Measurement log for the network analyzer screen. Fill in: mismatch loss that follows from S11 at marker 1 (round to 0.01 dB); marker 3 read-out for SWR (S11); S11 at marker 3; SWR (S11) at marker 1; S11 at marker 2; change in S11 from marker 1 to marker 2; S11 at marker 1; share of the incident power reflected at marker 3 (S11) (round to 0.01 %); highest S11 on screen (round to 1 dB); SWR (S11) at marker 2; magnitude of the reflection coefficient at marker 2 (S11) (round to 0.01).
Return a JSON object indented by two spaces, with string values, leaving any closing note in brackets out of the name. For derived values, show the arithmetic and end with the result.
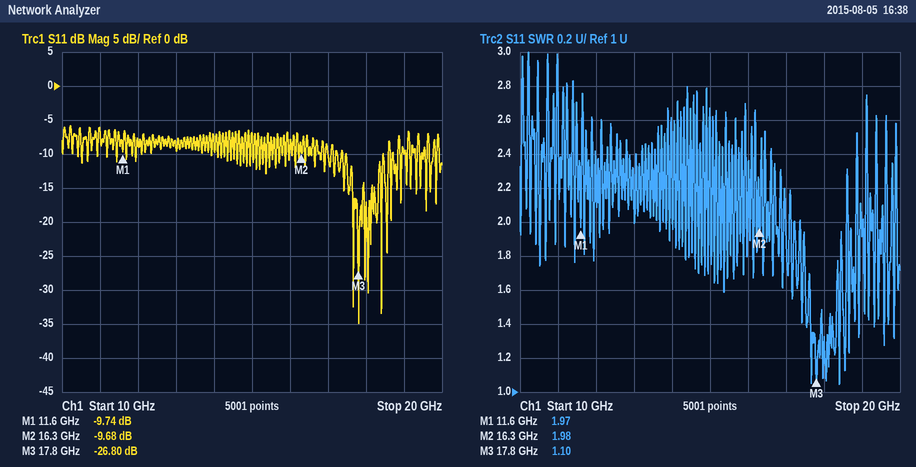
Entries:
{
  "mismatch loss that follows from S11 at marker 1": "−10 log10(1 − 10^(-9.74/10)) ≈ 0.49 dB",
  "marker 3 read-out for SWR": "1.10",
  "S11 at marker 3": "-26.80 dB",
  "SWR (S11) at marker 1": "1.97",
  "S11 at marker 2": "-9.68 dB",
  "change in S11 from marker 1 to marker 2": "-9.68 − (-9.74) = 0.06 dB",
  "S11 at marker 1": "-9.74 dB",
  "share of the incident power reflected at marker 3 (S11)": "10^(-26.8/10) ≈ 0.21 %",
  "highest S11 on screen": "-6 dB",
  "SWR (S11) at marker 2": "1.98",
  "magnitude of the reflection coefficient at marker 2 (S11)": "10^(-9.68/20) ≈ 0.33"
}
